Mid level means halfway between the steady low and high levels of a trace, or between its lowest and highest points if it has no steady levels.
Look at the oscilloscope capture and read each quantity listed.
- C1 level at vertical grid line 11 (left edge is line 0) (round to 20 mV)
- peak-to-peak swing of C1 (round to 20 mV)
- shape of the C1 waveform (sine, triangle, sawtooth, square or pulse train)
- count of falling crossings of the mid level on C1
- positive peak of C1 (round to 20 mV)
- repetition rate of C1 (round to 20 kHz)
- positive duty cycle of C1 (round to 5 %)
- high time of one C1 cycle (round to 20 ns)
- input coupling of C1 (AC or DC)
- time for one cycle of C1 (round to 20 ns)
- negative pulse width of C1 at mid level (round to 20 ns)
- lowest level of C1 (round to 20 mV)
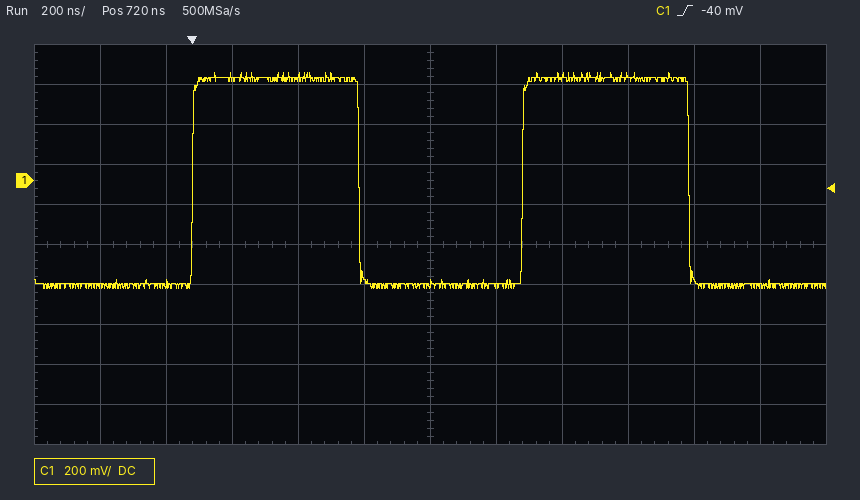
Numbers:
-520 mV
1.08 V
square
2
540 mV
1.00 MHz
50 %
500 ns
DC
1.00 µs
500 ns
-540 mV
